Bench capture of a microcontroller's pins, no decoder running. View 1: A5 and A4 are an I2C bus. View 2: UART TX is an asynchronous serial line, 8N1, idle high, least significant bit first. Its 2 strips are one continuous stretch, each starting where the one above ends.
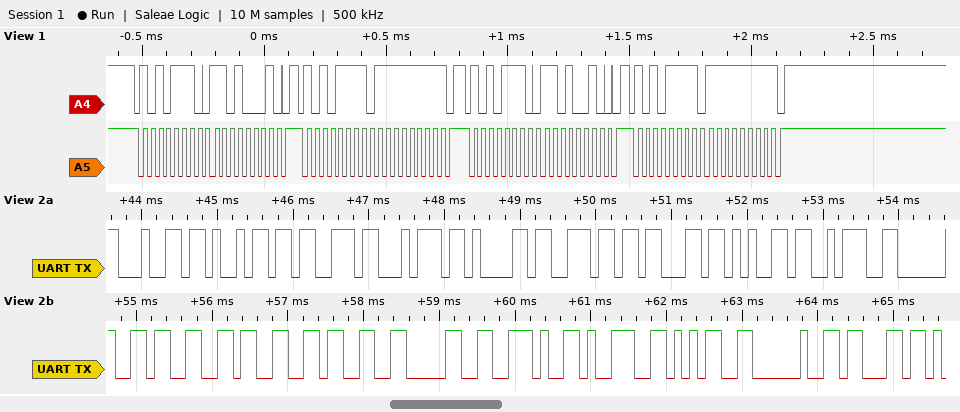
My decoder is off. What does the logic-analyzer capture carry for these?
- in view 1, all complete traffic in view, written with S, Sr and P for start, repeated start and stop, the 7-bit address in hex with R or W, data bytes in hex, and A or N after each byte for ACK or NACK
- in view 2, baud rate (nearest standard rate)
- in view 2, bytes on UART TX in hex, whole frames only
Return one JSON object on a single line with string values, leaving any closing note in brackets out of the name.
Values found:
{"in view 1, all complete traffic in view, written with S, Sr and P for start, repeated start and stop, the 7-bit address in hex with R or W, data bytes in hex, and A or N after each byte for ACK or NACK": "S 57W A D1 A P S 57R A FF N P S 57W A D2 A P S 57R A FF N P", "in view 2, baud rate": "9600 baud", "in view 2, bytes on UART TX in hex, whole frames only": "0x64 0x69 0x73 0x74 0x61 0x6E 0x63 0x65 0x3A 0x20 0x33 0x33 0x33 0x30 0x2E 0x39 0x35 0x20 0x63"}
